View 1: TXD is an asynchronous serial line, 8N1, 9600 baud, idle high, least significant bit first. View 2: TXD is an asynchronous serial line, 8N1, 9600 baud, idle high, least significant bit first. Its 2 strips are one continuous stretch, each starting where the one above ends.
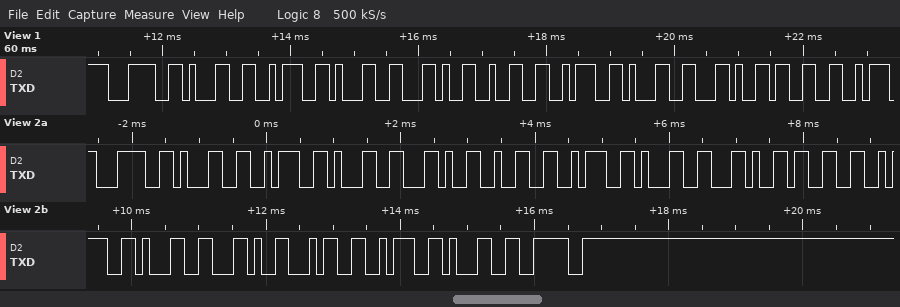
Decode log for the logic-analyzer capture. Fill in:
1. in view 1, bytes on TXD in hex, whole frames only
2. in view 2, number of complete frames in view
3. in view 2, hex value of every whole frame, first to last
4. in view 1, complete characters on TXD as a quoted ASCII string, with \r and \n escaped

0x3C 0x31 0x3A 0x31 0x2C 0x32 0x3A 0x31 0x2C 0x33
17
3C 31 3A 31 2C 32 3A 31 2C 33 3A 31 2C 34 3A 31 3E
"<1:1,2:1,3"
